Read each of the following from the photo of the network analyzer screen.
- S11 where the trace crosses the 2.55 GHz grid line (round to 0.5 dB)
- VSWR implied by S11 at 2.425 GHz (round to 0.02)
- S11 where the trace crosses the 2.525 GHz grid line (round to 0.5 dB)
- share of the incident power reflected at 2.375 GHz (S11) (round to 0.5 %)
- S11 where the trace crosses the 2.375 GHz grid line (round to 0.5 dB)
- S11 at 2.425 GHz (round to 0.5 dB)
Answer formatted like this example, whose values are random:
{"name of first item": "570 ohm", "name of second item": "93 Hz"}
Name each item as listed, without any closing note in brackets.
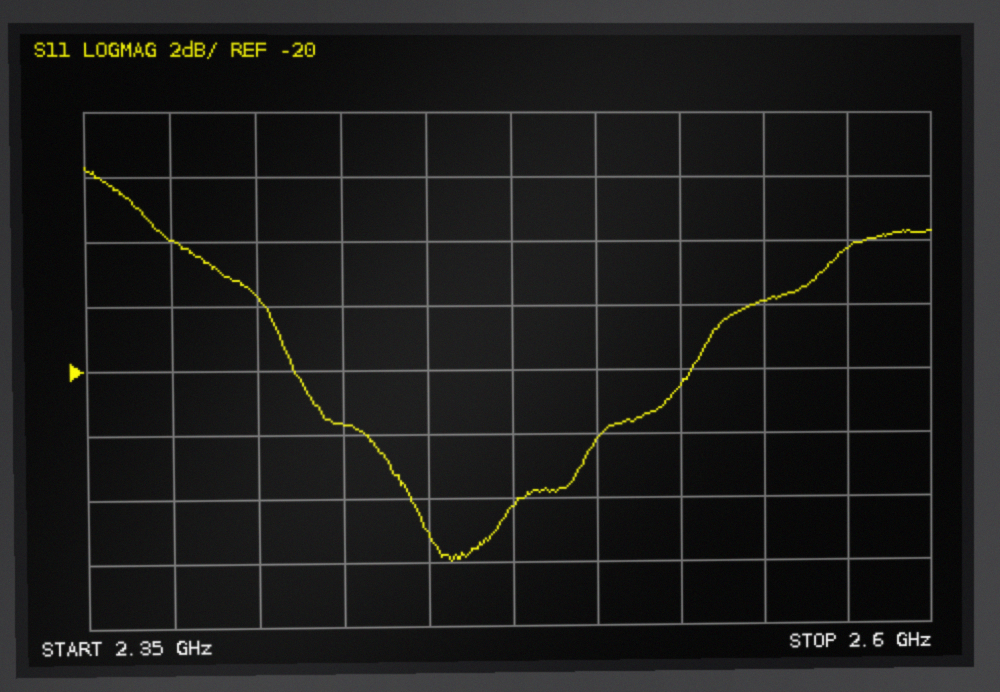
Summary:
{"S11 where the trace crosses the 2.55 GHz grid line": "-18.0 dB", "VSWR implied by S11 at 2.425 GHz": "1.18", "S11 where the trace crosses the 2.525 GHz grid line": "-20.5 dB", "share of the incident power reflected at 2.375 GHz (S11)": "2.5 %", "S11 where the trace crosses the 2.375 GHz grid line": "-16.0 dB", "S11 at 2.425 GHz": "-21.5 dB"}
